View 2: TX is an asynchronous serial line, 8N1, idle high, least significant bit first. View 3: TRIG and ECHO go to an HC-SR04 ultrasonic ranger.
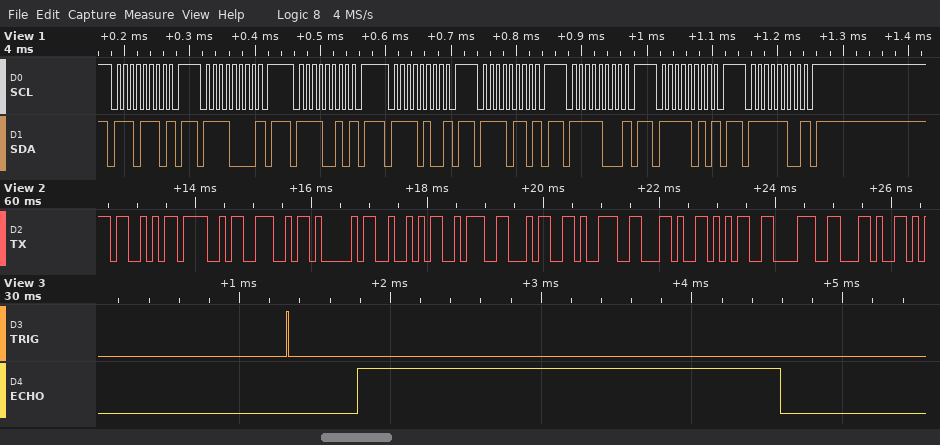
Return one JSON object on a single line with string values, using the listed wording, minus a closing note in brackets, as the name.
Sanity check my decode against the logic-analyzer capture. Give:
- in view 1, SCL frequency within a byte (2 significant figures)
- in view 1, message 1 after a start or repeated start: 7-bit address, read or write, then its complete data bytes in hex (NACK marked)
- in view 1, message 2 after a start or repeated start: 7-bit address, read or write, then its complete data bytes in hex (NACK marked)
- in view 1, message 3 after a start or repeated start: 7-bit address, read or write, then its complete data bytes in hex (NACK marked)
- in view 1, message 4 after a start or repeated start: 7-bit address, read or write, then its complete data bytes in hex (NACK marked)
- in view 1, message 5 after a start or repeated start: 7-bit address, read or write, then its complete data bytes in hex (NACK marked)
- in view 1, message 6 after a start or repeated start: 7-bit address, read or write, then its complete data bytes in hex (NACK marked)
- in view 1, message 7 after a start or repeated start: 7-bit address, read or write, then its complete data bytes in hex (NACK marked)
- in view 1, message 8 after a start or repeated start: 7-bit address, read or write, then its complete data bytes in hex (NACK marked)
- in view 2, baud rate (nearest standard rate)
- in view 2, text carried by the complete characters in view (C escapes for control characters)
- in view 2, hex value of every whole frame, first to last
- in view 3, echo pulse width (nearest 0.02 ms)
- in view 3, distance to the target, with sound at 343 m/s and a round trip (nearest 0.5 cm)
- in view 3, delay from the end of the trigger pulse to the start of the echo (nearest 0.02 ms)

{"in view 1, SCL frequency within a byte": "100 kHz", "in view 1, message 1 after a start or repeated start: 7-bit address, read or write, then its complete data bytes in hex": "0x77 write NACK", "in view 1, message 2 after a start or repeated start: 7-bit address, read or write, then its complete data bytes in hex": "0x78 write NACK", "in view 1, message 3 after a start or repeated start: 7-bit address, read or write, then its complete data bytes in hex": "0x79 write NACK", "in view 1, message 4 after a start or repeated start: 7-bit address, read or write, then its complete data bytes in hex": "0x7A write NACK", "in view 1, message 5 after a start or repeated start: 7-bit address, read or write, then its complete data bytes in hex": "0x7B write NACK", "in view 1, message 6 after a start or repeated start: 7-bit address, read or write, then its complete data bytes in hex": "0x7C write NACK", "in view 1, message 7 after a start or repeated start: 7-bit address, read or write, then its complete data bytes in hex": "0x7D write NACK", "in view 1, message 8 after a start or repeated start: 7-bit address, read or write, then its complete data bytes in hex": "0x7E write NACK", "in view 2, baud rate": "9600 baud", "in view 2, text carried by the complete characters in view": "\"SONAR:49,58,\"", "in view 2, hex value of every whole frame, first to last": "0x53 0x4F 0x4E 0x41 0x52 0x3A 0x34 0x39 0x2C 0x35 0x38 0x2C", "in view 3, echo pulse width": "2.80 ms", "in view 3, distance to the target, with sound at 343 m/s and a round trip": "48 cm", "in view 3, delay from the end of the trigger pulse to the start of the echo": "0.46 ms"}
